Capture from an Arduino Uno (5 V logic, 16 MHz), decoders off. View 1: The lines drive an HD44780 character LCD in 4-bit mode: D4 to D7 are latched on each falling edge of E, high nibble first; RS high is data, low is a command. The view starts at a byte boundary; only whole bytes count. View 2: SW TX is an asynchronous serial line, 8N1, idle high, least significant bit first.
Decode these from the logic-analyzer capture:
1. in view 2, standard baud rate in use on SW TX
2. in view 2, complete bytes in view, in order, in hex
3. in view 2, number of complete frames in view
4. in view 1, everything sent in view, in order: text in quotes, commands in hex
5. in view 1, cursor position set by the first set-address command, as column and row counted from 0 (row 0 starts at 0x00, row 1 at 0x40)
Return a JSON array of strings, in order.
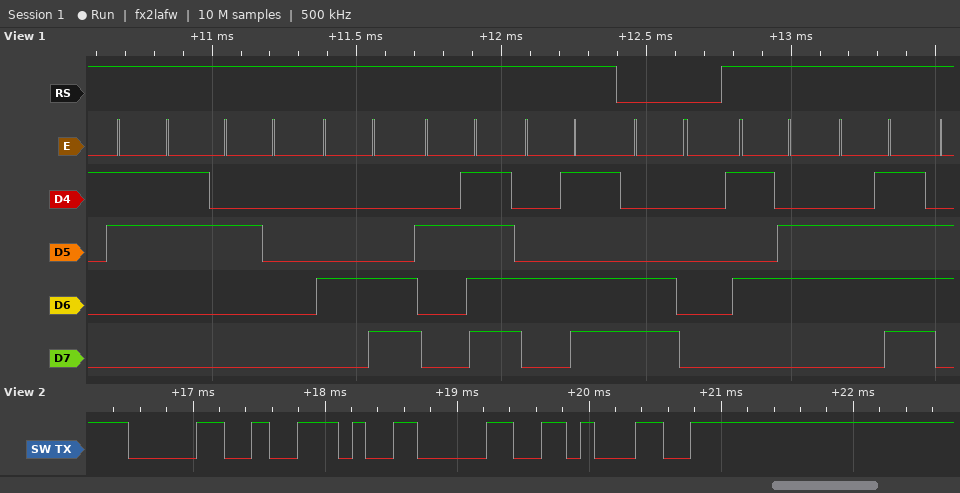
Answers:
["9600 baud", "30 2E 30 31", "4", "\"3 L/M\" 0xC0 \"Vo\"", "column 0, row 1"]
